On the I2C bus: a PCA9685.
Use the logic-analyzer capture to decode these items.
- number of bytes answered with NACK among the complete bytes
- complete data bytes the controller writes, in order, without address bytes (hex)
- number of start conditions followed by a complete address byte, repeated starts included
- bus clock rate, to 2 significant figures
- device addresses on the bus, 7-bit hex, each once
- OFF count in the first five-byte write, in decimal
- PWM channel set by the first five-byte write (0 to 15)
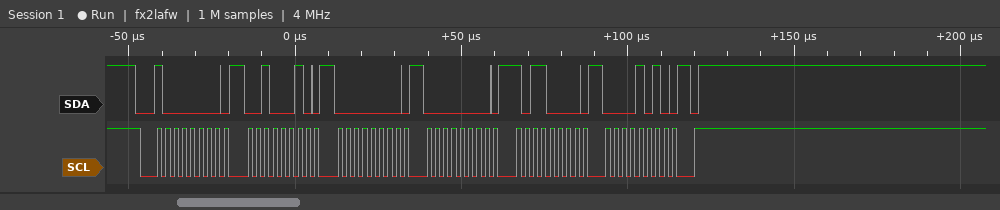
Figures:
0
22 00 00 B0 0A
1
400 kHz
0x40
2736
7
